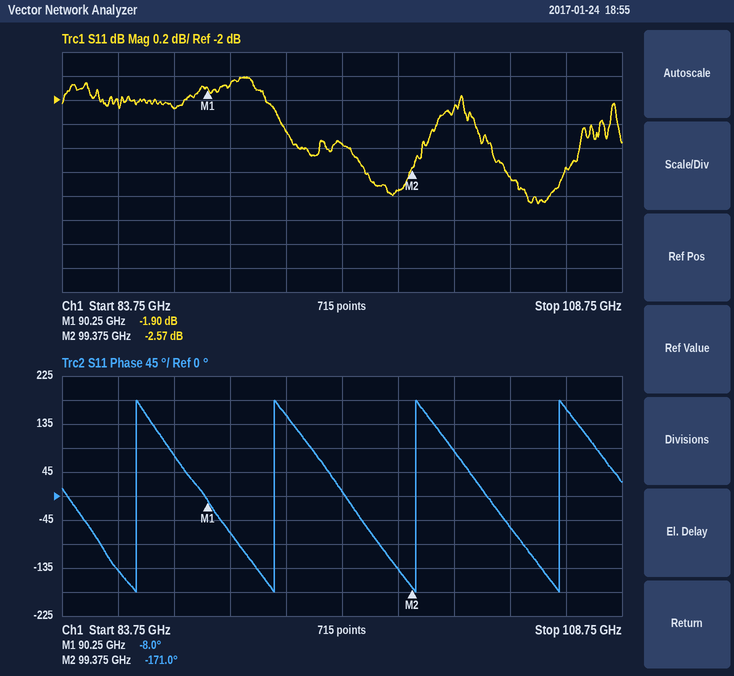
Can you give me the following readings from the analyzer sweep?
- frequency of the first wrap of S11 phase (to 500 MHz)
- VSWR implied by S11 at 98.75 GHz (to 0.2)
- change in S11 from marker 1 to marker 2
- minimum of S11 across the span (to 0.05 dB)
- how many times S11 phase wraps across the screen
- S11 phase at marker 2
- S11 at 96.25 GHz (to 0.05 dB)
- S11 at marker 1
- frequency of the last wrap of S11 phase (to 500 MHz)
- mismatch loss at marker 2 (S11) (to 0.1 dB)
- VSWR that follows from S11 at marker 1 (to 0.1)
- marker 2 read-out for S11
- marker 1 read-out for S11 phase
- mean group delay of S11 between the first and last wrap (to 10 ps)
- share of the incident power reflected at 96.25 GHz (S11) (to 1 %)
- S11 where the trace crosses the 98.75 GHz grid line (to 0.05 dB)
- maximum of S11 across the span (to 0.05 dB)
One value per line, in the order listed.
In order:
87.0 GHz
6.4
-0.67 dB
-2.85 dB
4
-171.0°
-2.35 dB
-1.90 dB
106.0 GHz
3.5 dB
9.2
-2.57 dB
-8.0°
160 ps
58 %
-2.75 dB
-1.80 dB
